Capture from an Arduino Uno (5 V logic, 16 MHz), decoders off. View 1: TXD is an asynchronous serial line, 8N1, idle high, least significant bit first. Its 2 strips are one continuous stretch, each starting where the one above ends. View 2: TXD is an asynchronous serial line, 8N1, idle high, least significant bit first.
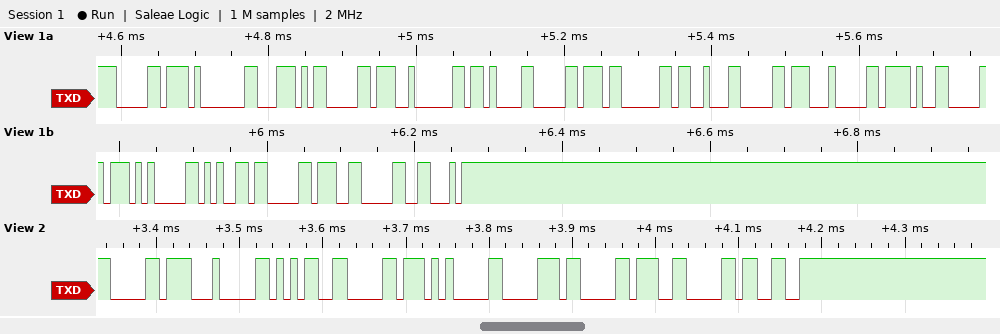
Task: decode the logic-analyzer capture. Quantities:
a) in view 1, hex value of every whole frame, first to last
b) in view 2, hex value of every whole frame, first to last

B0 01 5C B0 02 0B B0 03 13 B0 04 2F B0 05 65 B0 06 46
0xB0 0x04 0x35 0xB0 0x05 0x70 0xB0 0x06 0x33
